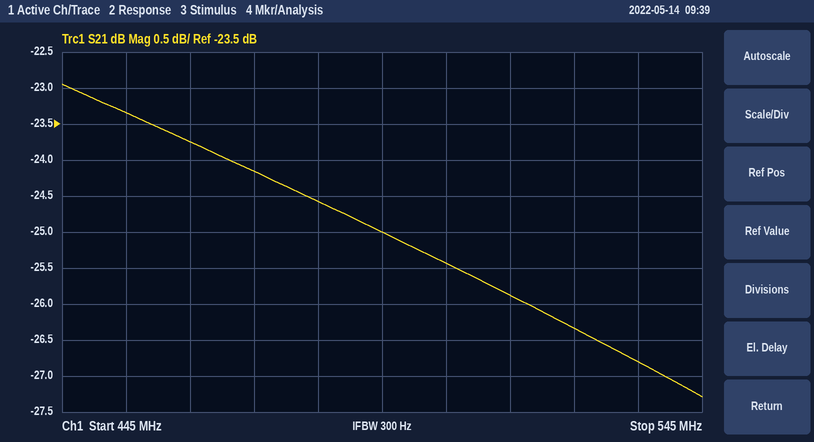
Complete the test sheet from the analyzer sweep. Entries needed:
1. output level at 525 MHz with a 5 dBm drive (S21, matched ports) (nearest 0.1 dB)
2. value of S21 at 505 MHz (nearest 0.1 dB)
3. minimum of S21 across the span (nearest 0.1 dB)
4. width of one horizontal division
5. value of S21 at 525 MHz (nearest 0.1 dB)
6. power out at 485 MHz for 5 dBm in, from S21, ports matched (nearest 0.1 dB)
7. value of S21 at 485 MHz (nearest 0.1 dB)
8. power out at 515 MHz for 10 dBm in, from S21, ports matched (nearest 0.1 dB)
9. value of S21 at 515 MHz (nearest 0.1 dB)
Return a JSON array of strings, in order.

["-21.3 dBm", "-25.4 dB", "-27.3 dB", "10 MHz", "-26.3 dB", "-19.6 dBm", "-24.6 dB", "-15.9 dBm", "-25.9 dB"]
